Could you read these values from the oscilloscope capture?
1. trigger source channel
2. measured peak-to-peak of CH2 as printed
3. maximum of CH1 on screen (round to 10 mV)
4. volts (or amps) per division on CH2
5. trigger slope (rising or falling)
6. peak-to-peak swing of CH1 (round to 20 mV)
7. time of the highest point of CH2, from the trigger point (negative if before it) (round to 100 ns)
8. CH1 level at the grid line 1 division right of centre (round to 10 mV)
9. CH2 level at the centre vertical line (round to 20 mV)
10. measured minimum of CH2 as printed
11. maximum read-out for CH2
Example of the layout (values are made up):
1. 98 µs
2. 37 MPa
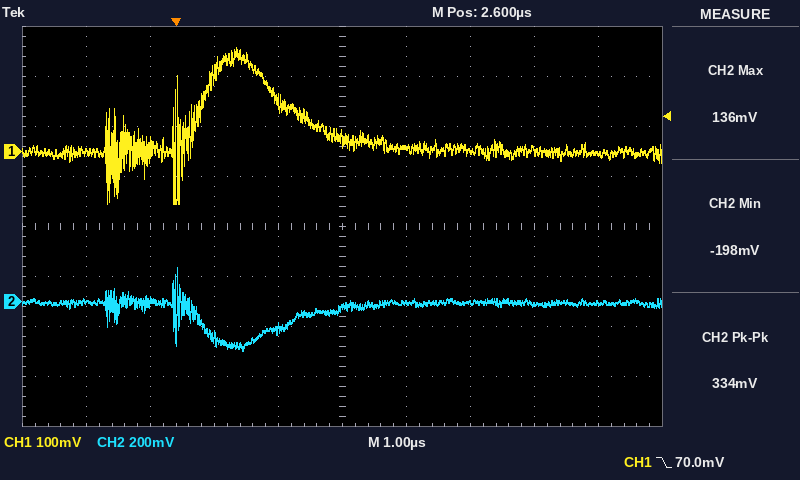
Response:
1. CH1
2. 334 mV
3. 210 mV
4. 200 mV
5. falling
6. 320 mV
7. 0.0 µs
8. 10 mV
9. -20 mV
10. -198 mV
11. 136 mV
